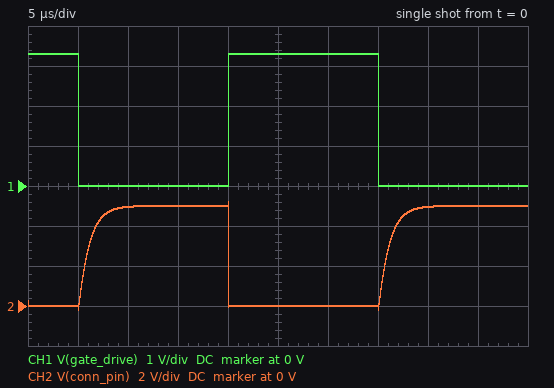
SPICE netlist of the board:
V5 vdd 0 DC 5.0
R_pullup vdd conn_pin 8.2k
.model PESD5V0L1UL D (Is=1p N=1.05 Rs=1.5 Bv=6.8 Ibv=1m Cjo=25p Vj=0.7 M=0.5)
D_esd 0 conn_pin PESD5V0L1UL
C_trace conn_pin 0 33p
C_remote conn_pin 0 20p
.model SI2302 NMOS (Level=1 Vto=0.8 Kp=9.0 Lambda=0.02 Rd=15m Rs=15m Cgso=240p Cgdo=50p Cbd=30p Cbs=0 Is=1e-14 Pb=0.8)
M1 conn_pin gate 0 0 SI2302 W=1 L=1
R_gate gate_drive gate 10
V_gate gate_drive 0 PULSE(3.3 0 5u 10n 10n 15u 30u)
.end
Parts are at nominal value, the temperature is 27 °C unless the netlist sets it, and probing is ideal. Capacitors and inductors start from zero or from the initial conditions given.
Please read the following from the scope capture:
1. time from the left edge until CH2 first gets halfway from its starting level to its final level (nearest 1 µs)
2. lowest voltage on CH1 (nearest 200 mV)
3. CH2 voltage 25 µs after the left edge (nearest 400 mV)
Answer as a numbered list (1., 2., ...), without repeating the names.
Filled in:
1. 6 µs
2. 0 V
3. 0 V
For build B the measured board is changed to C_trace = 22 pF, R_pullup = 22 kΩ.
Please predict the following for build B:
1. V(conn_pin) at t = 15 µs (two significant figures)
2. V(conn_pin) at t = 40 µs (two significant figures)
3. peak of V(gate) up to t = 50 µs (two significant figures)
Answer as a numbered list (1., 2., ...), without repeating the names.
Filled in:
1. 4.9 V
2. 4.2 V
3. 3.3 V
